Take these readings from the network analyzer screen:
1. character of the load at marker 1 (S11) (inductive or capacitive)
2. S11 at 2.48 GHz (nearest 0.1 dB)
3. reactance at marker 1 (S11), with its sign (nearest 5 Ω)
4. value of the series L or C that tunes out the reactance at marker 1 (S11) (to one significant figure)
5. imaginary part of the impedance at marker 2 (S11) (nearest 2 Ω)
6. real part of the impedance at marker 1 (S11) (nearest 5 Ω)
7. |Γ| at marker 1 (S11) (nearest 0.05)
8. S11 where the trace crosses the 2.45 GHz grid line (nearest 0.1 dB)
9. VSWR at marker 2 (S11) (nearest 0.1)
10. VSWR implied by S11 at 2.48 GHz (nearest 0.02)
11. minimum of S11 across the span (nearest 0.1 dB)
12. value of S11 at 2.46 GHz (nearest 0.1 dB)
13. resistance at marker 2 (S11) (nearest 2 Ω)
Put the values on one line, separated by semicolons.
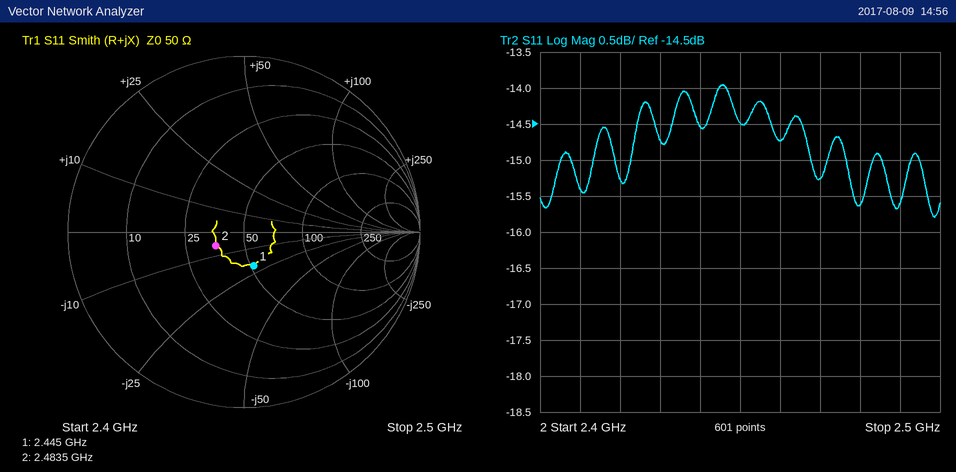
capacitive; -15.6 dB; -20 Ω; 1 nH; -6 Ω; 50 Ω; 0.20; -14.5 dB; 1.4; 1.40; -15.8 dB; -14.7 dB; 36 Ω
